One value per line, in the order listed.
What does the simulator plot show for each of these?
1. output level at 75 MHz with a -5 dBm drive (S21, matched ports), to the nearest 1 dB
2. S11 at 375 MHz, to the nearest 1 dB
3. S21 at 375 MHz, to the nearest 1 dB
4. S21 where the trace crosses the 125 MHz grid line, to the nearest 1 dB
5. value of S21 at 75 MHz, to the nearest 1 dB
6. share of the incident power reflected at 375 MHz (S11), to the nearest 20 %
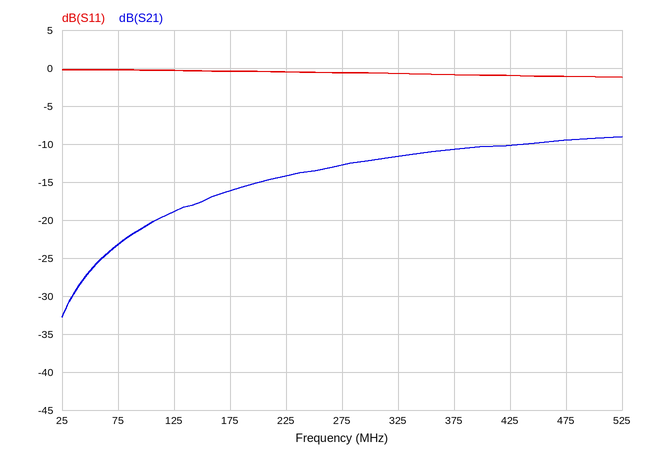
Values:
-28 dBm
-1 dB
-11 dB
-19 dB
-23 dB
80 %
